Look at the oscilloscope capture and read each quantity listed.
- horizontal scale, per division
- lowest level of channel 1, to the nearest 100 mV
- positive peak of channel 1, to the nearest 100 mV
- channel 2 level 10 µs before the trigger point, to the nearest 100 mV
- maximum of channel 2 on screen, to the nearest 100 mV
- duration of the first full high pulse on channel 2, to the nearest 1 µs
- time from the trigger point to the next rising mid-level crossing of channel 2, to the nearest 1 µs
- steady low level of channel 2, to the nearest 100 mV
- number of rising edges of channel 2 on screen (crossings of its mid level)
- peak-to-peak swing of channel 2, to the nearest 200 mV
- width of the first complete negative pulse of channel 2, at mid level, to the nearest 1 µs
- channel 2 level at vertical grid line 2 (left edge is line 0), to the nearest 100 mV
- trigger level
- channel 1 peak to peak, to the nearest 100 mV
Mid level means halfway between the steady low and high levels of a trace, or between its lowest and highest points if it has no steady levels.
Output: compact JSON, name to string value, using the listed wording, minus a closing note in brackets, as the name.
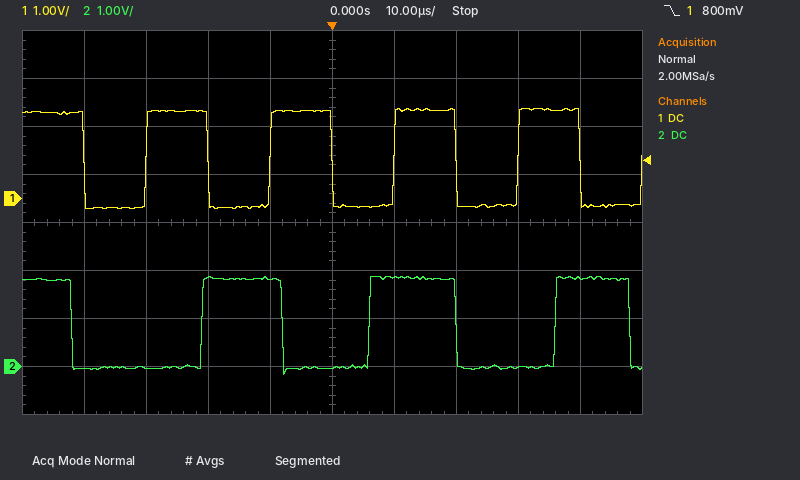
{"horizontal scale, per division": "10 µs", "lowest level of channel 1, to the nearest 100 mV": "-200 mV", "positive peak of channel 1, to the nearest 100 mV": "1.9 V", "channel 2 level 10 µs before the trigger point, to the nearest 100 mV": "1.8 V", "maximum of channel 2 on screen, to the nearest 100 mV": "1.9 V", "duration of the first full high pulse on channel 2, to the nearest 1 µs": "13 µs", "time from the trigger point to the next rising mid-level crossing of channel 2, to the nearest 1 µs": "6 µs", "steady low level of channel 2, to the nearest 100 mV": "0.0 V", "number of rising edges of channel 2 on screen": "3", "peak-to-peak swing of channel 2, to the nearest 200 mV": "2.0 V", "width of the first complete negative pulse of channel 2, at mid level, to the nearest 1 µs": "21 µs", "channel 2 level at vertical grid line 2 (left edge is line 0), to the nearest 100 mV": "0.0 V", "trigger level": "800 mV", "channel 1 peak to peak, to the nearest 100 mV": "2.1 V"}
